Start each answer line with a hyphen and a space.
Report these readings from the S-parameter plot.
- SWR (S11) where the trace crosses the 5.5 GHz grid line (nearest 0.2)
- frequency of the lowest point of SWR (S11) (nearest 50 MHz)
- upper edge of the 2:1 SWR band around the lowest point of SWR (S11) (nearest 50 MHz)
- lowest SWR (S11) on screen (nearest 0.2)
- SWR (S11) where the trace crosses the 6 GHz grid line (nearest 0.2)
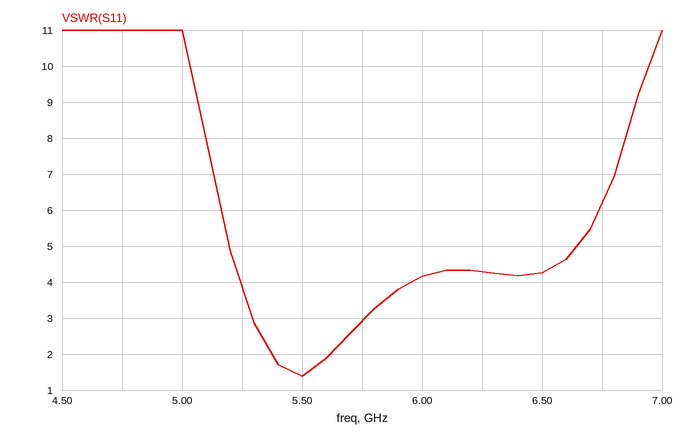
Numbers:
- 1.4
- 5.50 GHz
- 5.60 GHz
- 1.4
- 4.2
